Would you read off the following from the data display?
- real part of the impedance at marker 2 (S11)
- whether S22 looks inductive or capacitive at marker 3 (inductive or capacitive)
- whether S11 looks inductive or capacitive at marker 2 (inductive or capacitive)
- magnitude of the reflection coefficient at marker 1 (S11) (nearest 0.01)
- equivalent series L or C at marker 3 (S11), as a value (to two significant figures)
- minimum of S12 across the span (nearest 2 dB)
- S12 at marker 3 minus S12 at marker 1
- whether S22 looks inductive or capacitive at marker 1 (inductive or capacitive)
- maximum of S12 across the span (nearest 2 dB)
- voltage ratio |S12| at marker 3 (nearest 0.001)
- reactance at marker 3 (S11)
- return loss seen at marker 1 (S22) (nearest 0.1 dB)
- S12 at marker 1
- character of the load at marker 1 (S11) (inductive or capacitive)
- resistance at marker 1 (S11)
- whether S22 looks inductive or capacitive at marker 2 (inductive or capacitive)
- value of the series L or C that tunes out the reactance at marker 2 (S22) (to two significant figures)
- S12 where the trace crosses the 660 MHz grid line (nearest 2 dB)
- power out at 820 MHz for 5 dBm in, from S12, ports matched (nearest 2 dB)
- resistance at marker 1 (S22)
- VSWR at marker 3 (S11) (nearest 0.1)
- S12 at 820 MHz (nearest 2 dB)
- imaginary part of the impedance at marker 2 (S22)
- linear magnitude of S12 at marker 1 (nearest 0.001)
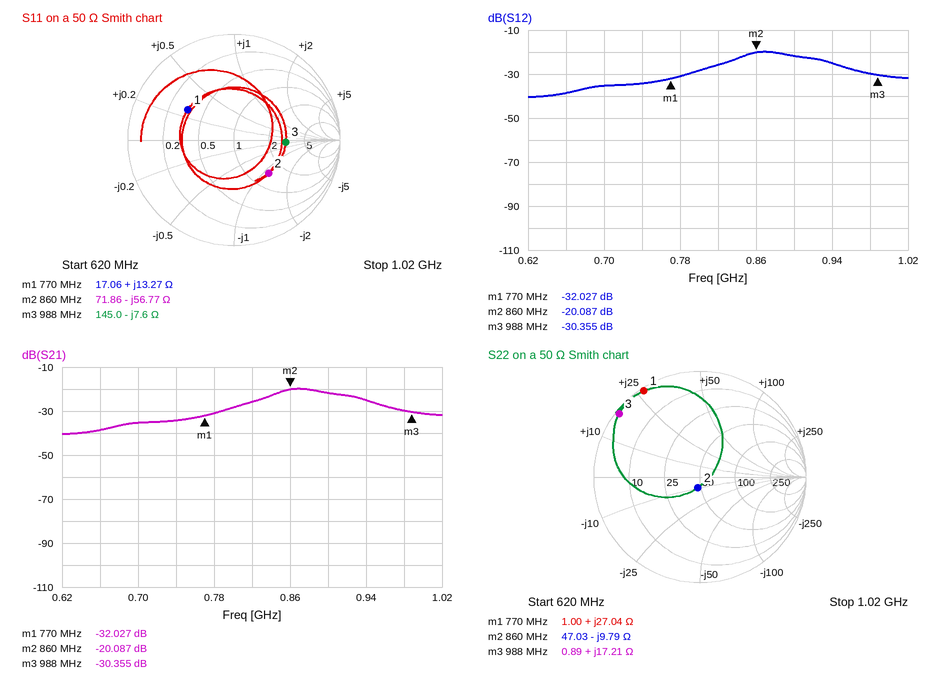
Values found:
71.86 Ω
inductive
capacitive
0.52
21 pF
-40 dB
1.672 dB
inductive
-20 dB
0.030
-7.6 Ω
0.3 dB
-32.027 dB
inductive
17.06 Ω
capacitive
1.8 nH
-38 dB
-20 dBm
1.00 Ω
2.9
-26 dB
-9.79 Ω
0.025
